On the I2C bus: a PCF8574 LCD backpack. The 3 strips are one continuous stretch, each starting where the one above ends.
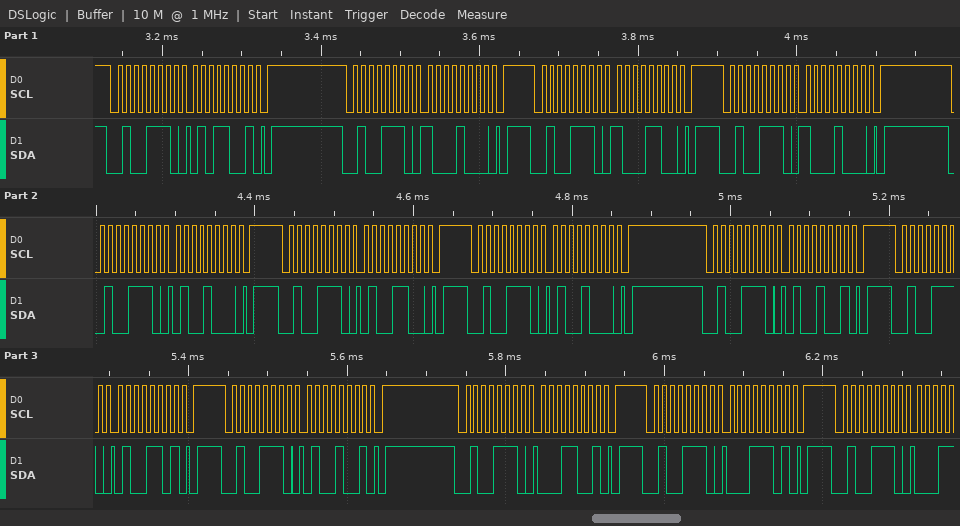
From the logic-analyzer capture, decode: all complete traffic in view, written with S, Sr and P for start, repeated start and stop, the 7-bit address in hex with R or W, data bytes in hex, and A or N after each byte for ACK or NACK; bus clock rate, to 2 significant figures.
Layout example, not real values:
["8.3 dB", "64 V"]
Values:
["S 27W A 59 A P S 27W A 88 A P S 27W A 8C A P S 27W A 88 A P S 27W A 48 A P S 27W A 4C A P S 27W A 48 A P S 27W A 49 A P S 27W A 4D A P S 27W A 49 A P S 27W A 19 A P S 27W A 1D A P S 27W A", "100 kHz"]
